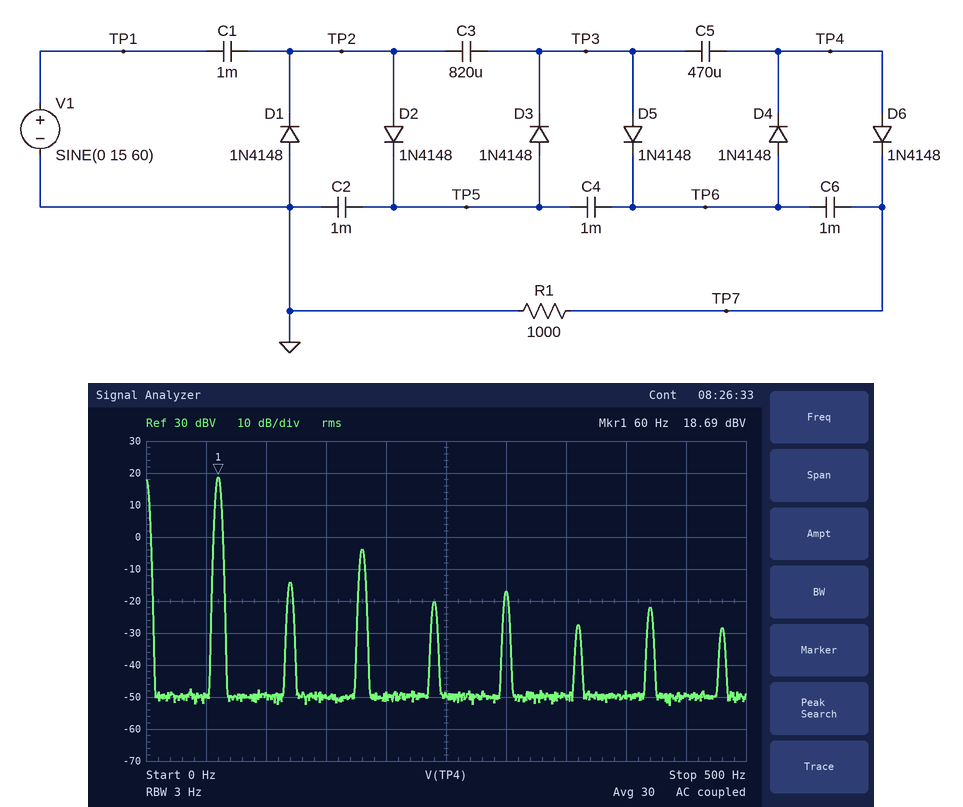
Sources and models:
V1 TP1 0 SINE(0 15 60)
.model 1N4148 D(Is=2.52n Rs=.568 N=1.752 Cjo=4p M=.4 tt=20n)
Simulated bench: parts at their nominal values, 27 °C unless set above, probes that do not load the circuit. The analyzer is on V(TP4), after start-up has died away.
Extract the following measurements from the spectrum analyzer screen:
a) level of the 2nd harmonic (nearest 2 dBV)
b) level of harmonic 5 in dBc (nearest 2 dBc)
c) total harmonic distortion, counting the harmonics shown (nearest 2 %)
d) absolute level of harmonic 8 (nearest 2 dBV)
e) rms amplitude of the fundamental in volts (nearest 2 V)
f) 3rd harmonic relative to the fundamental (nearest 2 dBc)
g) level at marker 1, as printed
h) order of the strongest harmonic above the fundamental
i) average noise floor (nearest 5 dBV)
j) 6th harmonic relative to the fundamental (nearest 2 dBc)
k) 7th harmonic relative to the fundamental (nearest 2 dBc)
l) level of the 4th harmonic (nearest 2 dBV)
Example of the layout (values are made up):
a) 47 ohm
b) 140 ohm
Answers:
a) -14 dBV
b) -36 dBc
c) 8 %
d) -28 dBV
e) 8 V
f) -22 dBc
g) 18.69 dBV
h) 3
i) -50 dBV
j) -46 dBc
k) -40 dBc
l) -20 dBV
